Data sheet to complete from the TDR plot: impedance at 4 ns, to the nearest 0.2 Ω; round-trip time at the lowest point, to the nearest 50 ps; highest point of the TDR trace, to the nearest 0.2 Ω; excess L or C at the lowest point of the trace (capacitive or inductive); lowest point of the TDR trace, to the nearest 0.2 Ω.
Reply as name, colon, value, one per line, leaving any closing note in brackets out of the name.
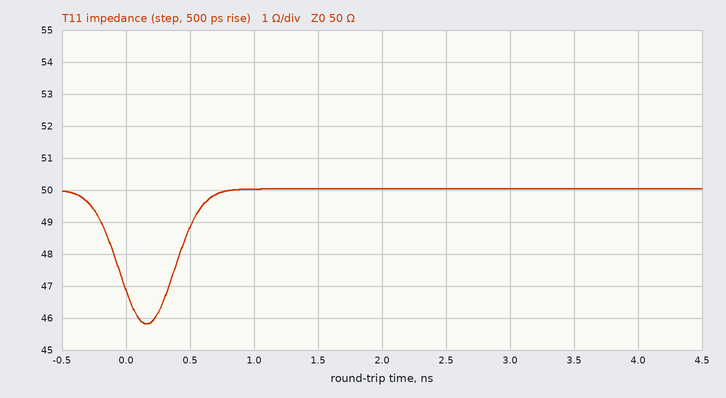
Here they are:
impedance at 4 ns, to the nearest 0.2 Ω: 50.0 Ω
round-trip time at the lowest point, to the nearest 50 ps: 150 ps
highest point of the TDR trace, to the nearest 0.2 Ω: 50.0 Ω
excess L or C at the lowest point of the trace: capacitive
lowest point of the TDR trace, to the nearest 0.2 Ω: 45.8 Ω
